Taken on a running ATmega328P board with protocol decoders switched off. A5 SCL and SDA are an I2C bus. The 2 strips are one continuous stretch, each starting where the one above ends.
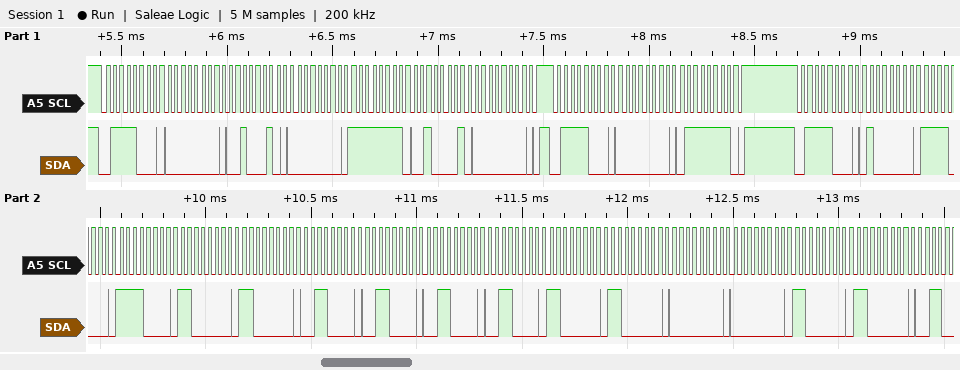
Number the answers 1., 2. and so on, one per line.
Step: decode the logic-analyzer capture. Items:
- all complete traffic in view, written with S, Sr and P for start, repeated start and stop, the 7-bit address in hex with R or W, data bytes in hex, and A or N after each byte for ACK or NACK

1. S 3CW A 00 A 22 A 00 A FF A 21 A 00 A P S 3CW A 00 A 7F A P S 3CW A 40 A F0 A F0 A C0 A C0 A 30 A 30 A 30 A 30 A C0 A C0 A 00 A 00 A C0 A C0 A
